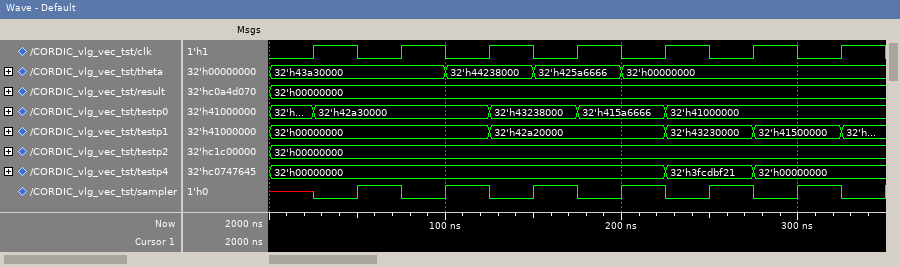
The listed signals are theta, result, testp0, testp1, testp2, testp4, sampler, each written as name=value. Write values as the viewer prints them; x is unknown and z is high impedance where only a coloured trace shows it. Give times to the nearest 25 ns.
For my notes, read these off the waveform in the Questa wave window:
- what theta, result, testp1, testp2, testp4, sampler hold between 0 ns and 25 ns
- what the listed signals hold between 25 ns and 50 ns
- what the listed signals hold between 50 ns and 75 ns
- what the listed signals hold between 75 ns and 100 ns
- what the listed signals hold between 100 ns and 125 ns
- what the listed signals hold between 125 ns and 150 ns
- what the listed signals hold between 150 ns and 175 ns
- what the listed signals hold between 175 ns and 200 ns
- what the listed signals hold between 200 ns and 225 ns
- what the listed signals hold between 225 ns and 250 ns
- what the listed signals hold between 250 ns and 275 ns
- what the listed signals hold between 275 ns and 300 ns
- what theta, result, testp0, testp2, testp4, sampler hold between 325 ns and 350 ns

theta=32'h43a30000, result=32'h00000000, testp1=32'h00000000, testp2=32'h00000000, testp4=32'h00000000, sampler=x
theta=32'h43a30000, result=32'h00000000, testp0=32'h42a30000, testp1=32'h00000000, testp2=32'h00000000, testp4=32'h00000000, sampler=0
theta=32'h43a30000, result=32'h00000000, testp0=32'h42a30000, testp1=32'h00000000, testp2=32'h00000000, testp4=32'h00000000, sampler=1
theta=32'h43a30000, result=32'h00000000, testp0=32'h42a30000, testp1=32'h00000000, testp2=32'h00000000, testp4=32'h00000000, sampler=0
theta=32'h44238000, result=32'h00000000, testp0=32'h42a30000, testp1=32'h00000000, testp2=32'h00000000, testp4=32'h00000000, sampler=1
theta=32'h44238000, result=32'h00000000, testp0=32'h43238000, testp1=32'h42a20000, testp2=32'h00000000, testp4=32'h00000000, sampler=0
theta=32'h425a6666, result=32'h00000000, testp0=32'h43238000, testp1=32'h42a20000, testp2=32'h00000000, testp4=32'h00000000, sampler=1
theta=32'h425a6666, result=32'h00000000, testp0=32'h415a6666, testp1=32'h42a20000, testp2=32'h00000000, testp4=32'h00000000, sampler=0
theta=32'h00000000, result=32'h00000000, testp0=32'h415a6666, testp1=32'h42a20000, testp2=32'h00000000, testp4=32'h00000000, sampler=1
theta=32'h00000000, result=32'h00000000, testp0=32'h41000000, testp1=32'h43230000, testp2=32'h00000000, testp4=32'h3fcdbf21, sampler=0
theta=32'h00000000, result=32'h00000000, testp0=32'h41000000, testp1=32'h43230000, testp2=32'h00000000, testp4=32'h3fcdbf21, sampler=1
theta=32'h00000000, result=32'h00000000, testp0=32'h41000000, testp1=32'h41500000, testp2=32'h00000000, testp4=32'h00000000, sampler=0
theta=32'h00000000, result=32'h00000000, testp0=32'h41000000, testp2=32'h00000000, testp4=32'h00000000, sampler=0
